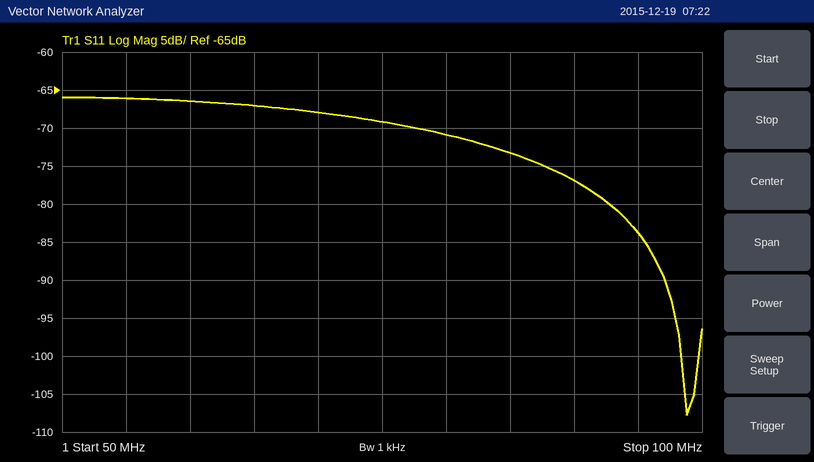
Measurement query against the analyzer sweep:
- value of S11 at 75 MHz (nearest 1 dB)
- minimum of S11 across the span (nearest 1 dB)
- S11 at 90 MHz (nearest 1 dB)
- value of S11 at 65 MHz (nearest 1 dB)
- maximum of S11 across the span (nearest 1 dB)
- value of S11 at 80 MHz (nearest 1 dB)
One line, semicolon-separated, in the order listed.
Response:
-69 dB; -108 dB; -77 dB; -67 dB; -66 dB; -71 dB
